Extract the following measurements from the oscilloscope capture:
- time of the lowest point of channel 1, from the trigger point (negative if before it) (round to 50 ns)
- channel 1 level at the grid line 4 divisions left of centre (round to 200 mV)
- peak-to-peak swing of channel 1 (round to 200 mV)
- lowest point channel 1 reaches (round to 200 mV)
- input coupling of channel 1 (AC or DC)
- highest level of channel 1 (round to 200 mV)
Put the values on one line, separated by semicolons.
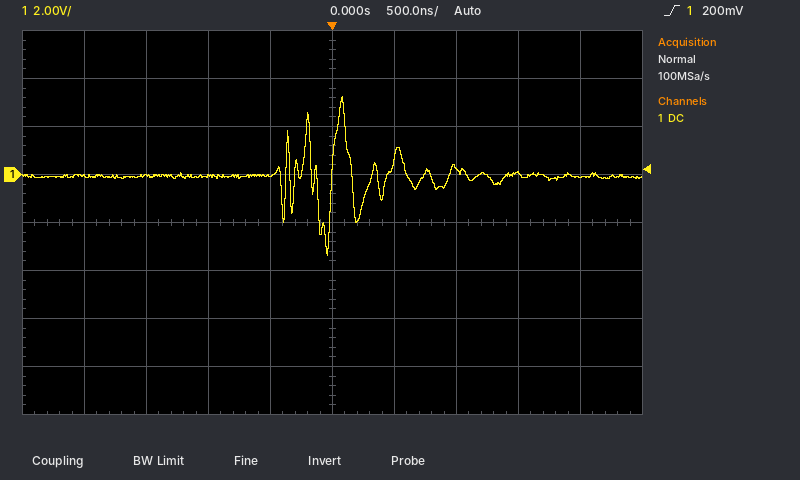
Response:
-50 ns; 0.0 V; 6.6 V; -3.4 V; DC; 3.2 V
